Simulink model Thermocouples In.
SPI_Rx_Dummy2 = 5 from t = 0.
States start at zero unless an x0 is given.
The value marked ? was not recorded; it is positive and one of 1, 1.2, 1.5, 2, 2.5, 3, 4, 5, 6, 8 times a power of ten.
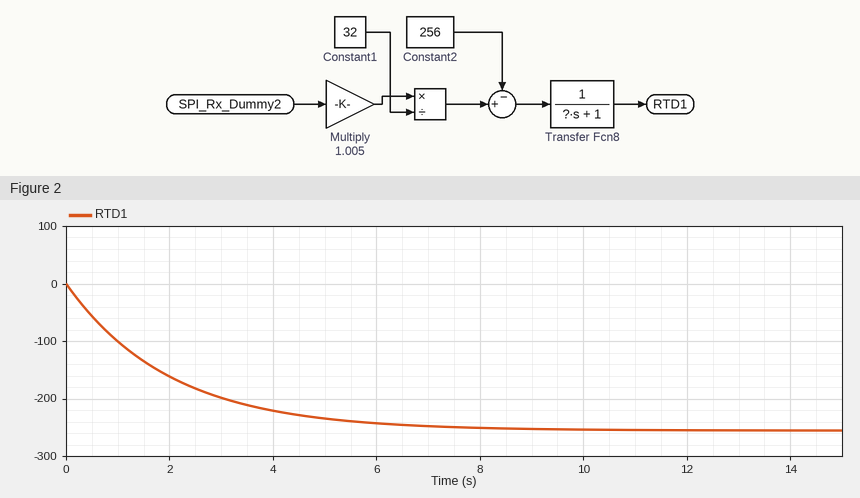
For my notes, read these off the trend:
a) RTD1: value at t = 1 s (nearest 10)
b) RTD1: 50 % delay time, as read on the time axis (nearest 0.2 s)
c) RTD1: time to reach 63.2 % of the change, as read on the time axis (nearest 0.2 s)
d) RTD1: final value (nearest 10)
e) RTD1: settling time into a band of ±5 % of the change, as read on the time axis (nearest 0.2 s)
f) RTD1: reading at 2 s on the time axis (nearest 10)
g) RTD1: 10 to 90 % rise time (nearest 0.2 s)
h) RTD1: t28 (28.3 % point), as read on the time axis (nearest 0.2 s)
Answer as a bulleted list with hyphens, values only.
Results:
- -100
- 1.4 s
- 2.0 s
- -260
- 6.0 s
- -160
- 4.4 s
- 0.6 s
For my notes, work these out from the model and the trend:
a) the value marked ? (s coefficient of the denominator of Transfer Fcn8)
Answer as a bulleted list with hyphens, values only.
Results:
- 2
